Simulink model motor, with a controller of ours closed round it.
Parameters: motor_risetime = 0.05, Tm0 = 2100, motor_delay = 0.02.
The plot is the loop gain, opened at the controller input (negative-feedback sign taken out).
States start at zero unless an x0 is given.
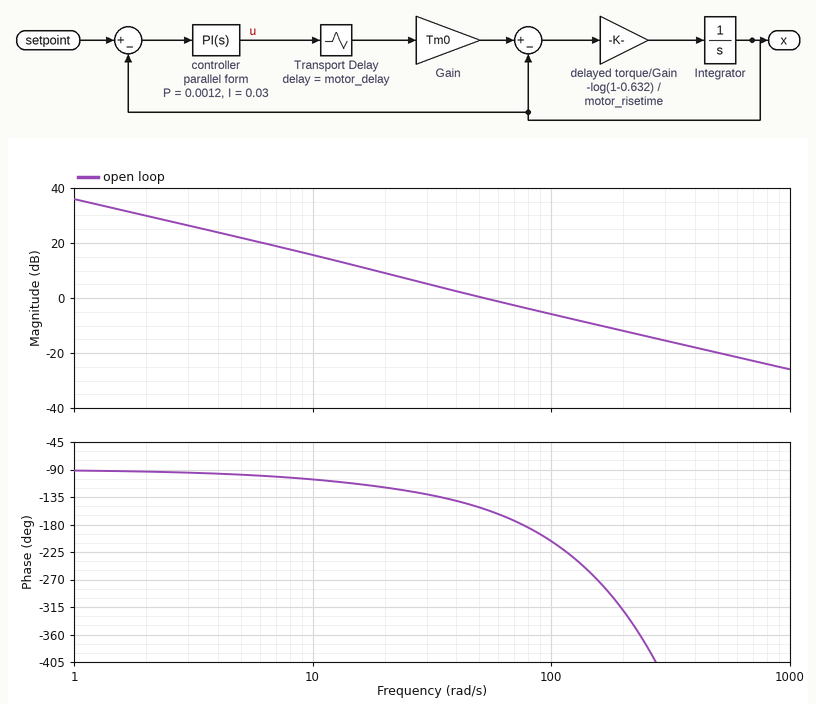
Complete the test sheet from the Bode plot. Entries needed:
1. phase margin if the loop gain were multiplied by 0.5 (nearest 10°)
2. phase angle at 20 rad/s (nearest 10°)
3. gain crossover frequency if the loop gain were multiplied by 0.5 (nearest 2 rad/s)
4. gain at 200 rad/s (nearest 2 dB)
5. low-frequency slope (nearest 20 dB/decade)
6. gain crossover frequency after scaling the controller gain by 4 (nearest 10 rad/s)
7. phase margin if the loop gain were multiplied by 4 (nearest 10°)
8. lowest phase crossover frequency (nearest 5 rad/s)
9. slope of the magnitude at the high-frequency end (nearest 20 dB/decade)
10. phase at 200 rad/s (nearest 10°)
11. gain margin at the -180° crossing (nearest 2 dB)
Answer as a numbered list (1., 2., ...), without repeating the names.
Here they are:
1. 50°
2. -120°
3. 28 rad/s
4. -12 dB
5. -20 dB/decade
6. 200 rad/s
7. -140°
8. 75 rad/s
9. -20 dB/decade
10. -320°
11. 4 dB
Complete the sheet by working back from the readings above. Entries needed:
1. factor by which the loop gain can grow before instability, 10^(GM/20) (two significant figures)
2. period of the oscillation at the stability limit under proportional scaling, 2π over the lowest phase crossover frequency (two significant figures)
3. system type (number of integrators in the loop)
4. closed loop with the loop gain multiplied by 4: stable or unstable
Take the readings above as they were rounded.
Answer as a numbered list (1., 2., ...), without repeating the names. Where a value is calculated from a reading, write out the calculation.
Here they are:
1. 10^(4 / 20) = 1.6
2. 2π / 75 = 0.084 s
3. 1
4. unstable
